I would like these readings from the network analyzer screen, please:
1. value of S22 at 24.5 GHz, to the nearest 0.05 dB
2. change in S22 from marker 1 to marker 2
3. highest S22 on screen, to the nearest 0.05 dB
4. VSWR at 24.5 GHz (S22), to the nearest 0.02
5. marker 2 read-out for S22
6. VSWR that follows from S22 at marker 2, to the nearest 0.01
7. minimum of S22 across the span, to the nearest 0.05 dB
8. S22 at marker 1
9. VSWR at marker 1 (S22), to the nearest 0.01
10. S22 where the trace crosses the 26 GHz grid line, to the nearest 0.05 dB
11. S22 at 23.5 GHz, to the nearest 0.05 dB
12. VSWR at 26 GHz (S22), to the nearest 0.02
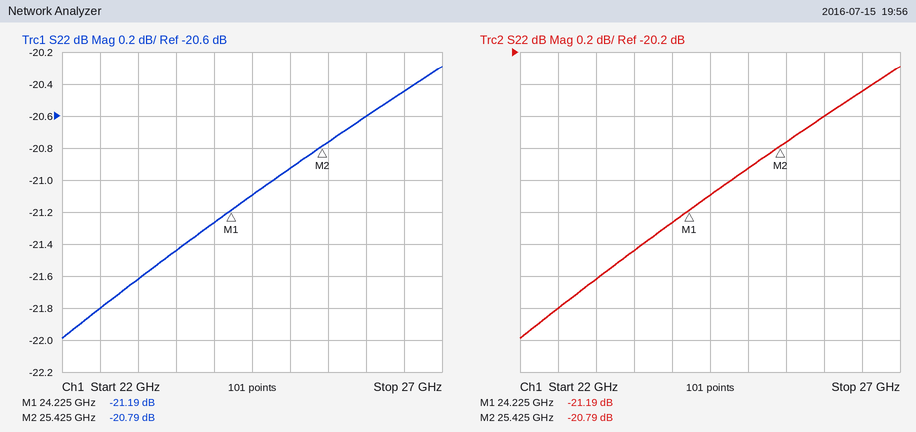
-21.10 dB
0.40 dB
-20.30 dB
1.20
-20.79 dB
1.20
-22.00 dB
-21.19 dB
1.19
-20.60 dB
-21.45 dB
1.20
